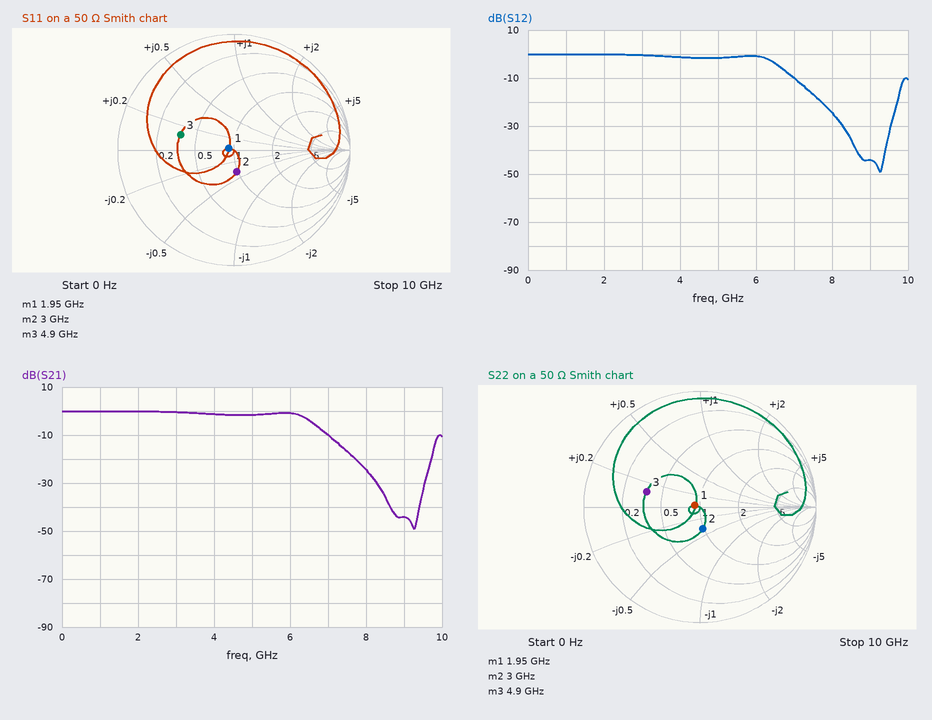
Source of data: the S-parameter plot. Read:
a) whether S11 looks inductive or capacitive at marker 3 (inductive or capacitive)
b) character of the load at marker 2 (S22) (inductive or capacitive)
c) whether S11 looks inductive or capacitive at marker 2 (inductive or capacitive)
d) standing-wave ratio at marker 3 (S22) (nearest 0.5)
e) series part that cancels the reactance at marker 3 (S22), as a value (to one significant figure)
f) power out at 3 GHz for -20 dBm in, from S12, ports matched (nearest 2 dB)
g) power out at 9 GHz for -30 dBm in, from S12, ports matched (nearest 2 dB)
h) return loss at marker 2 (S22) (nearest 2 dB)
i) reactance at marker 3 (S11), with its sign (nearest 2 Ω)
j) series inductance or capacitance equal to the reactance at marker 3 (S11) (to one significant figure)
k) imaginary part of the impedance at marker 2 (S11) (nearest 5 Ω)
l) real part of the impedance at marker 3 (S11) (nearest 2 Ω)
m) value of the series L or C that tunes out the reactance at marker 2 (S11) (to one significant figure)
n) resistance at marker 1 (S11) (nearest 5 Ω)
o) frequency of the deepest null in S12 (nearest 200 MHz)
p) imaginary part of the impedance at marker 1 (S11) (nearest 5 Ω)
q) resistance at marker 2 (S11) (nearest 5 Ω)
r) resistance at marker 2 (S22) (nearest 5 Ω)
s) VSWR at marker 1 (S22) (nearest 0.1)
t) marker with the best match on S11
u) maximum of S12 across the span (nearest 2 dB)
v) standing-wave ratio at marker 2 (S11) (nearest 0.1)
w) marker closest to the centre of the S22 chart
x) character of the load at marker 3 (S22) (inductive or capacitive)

inductive
capacitive
capacitive
3.0
5 pF
-20 dBm
-74 dBm
14 dB
+6 Ω
200 pH
-20 Ω
18 Ω
1 nH
45 Ω
9.2 GHz
0 Ω
50 Ω
50 Ω
1.1
marker 1
0 dB
1.5
marker 1
inductive
